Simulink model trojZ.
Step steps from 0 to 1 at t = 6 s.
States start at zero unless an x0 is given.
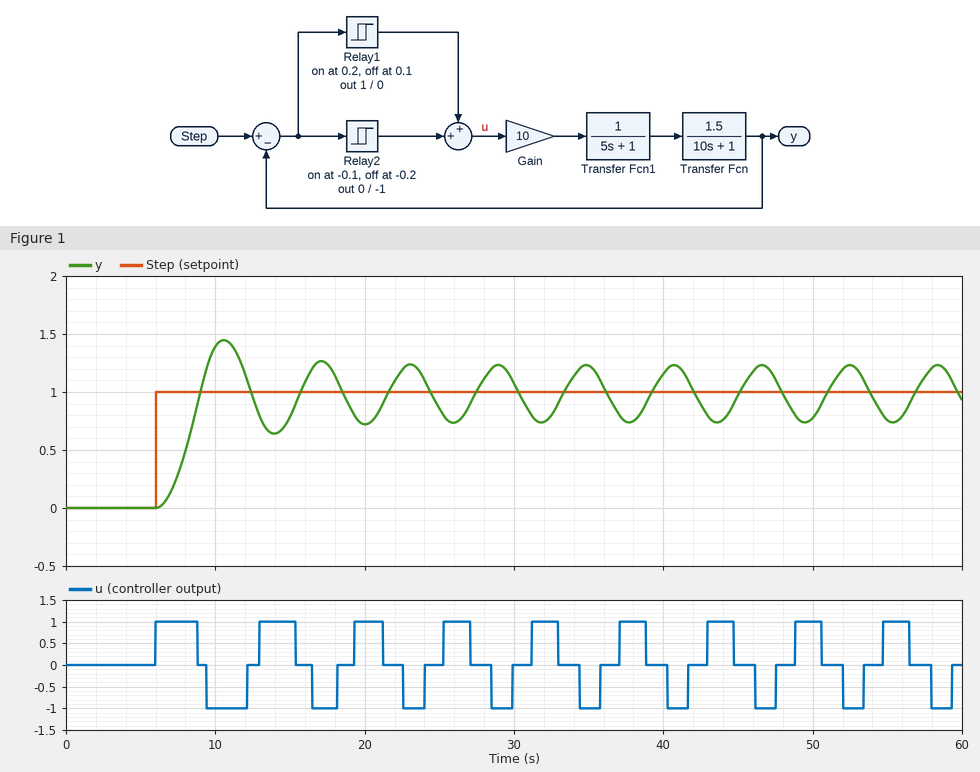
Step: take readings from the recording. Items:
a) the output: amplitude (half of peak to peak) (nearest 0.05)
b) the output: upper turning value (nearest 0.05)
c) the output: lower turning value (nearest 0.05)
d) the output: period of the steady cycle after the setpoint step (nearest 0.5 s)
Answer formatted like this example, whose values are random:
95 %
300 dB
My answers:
0.25
1.25
0.75
6.0 s
